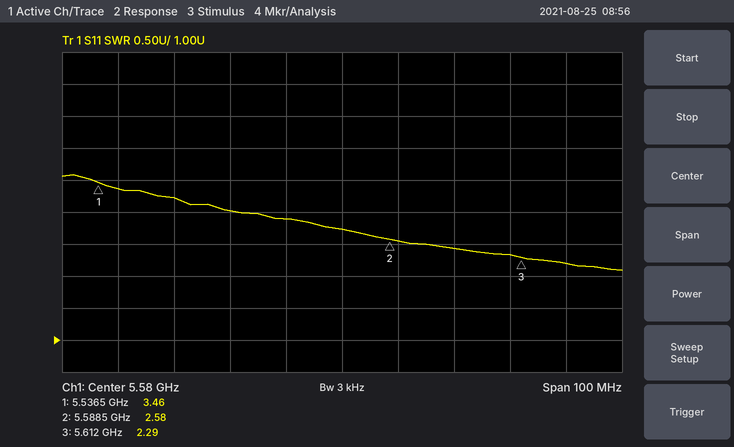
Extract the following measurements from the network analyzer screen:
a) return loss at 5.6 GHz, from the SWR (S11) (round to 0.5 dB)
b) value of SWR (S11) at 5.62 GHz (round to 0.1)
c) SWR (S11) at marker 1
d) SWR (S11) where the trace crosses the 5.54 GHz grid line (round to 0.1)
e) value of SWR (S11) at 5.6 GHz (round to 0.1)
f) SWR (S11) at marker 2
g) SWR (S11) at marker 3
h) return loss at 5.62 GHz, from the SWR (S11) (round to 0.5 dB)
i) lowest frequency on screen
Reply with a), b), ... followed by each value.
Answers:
a) 7.5 dB
b) 2.2
c) 3.46
d) 3.4
e) 2.4
f) 2.58
g) 2.29
h) 8.5 dB
i) 5.53 GHz
